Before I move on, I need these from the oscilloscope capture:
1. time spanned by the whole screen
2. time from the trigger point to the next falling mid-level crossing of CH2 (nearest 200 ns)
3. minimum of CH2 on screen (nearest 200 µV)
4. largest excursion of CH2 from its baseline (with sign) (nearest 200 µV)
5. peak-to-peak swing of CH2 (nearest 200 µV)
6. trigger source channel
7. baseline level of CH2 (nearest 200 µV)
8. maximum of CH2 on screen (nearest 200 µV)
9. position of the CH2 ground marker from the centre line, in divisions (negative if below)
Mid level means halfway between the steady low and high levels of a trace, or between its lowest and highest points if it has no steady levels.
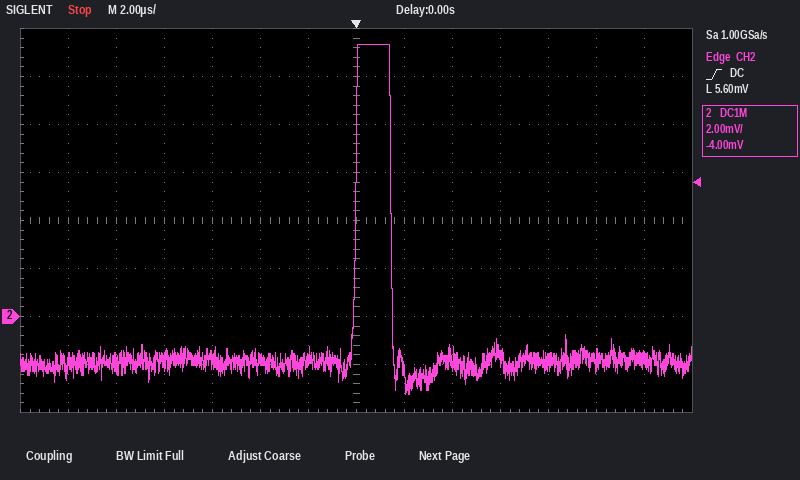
28 µs
1.4 µs
-3.2 mV
+13.2 mV
14.6 mV
CH2
-1.8 mV
11.4 mV
-2.0 div
